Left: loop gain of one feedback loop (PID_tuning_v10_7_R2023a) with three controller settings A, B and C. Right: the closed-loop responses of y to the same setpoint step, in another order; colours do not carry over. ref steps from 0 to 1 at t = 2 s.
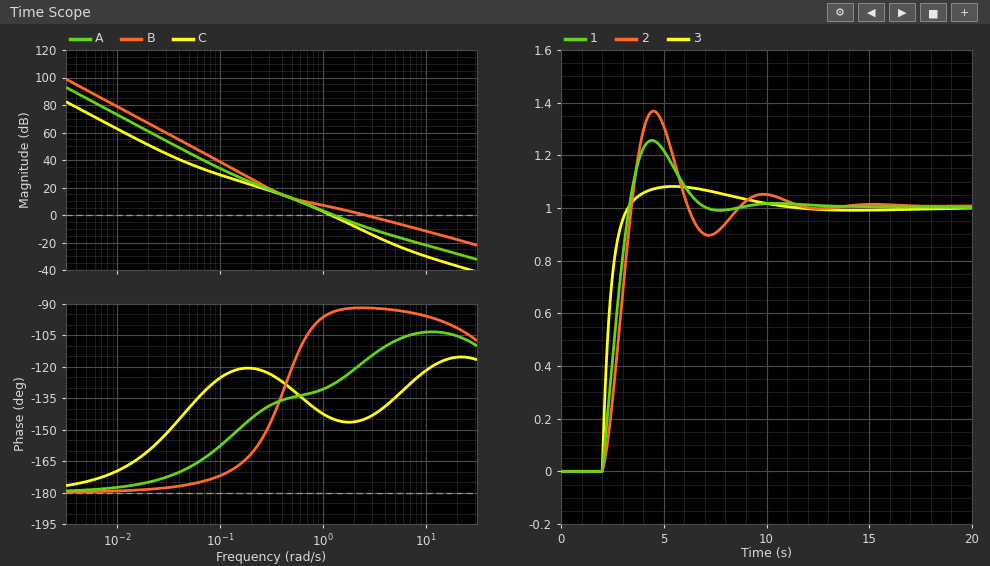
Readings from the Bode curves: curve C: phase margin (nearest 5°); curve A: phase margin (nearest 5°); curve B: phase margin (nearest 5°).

35°
50°
90°
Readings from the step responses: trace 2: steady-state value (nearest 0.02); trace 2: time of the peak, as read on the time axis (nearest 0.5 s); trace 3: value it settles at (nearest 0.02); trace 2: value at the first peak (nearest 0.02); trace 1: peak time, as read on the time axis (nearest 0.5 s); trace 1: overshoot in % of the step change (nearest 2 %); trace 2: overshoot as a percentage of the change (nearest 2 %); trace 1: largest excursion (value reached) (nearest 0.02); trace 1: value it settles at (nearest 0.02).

1.00
4.5 s
1.00
1.36
4.5 s
26 %
36 %
1.26
1.00
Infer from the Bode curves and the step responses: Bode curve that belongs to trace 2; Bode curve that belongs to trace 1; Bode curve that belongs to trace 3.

C
A
B
